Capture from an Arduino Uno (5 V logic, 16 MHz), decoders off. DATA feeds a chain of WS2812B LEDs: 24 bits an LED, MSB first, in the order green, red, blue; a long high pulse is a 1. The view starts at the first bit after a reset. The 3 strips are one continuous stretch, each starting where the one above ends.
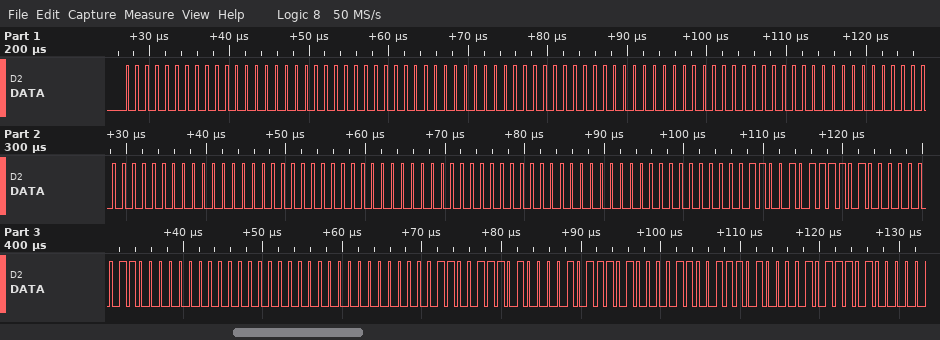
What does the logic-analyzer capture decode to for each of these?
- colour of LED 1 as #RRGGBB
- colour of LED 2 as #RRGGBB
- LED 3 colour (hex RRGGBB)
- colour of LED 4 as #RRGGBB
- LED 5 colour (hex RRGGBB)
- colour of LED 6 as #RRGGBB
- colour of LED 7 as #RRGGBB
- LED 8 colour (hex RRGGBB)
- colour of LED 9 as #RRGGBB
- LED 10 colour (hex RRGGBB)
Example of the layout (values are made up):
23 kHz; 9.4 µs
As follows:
#000000; #000000; #000000; #000000; #000000; #000000; #E8650C; #000000; #E80C5D; #E80C5D
